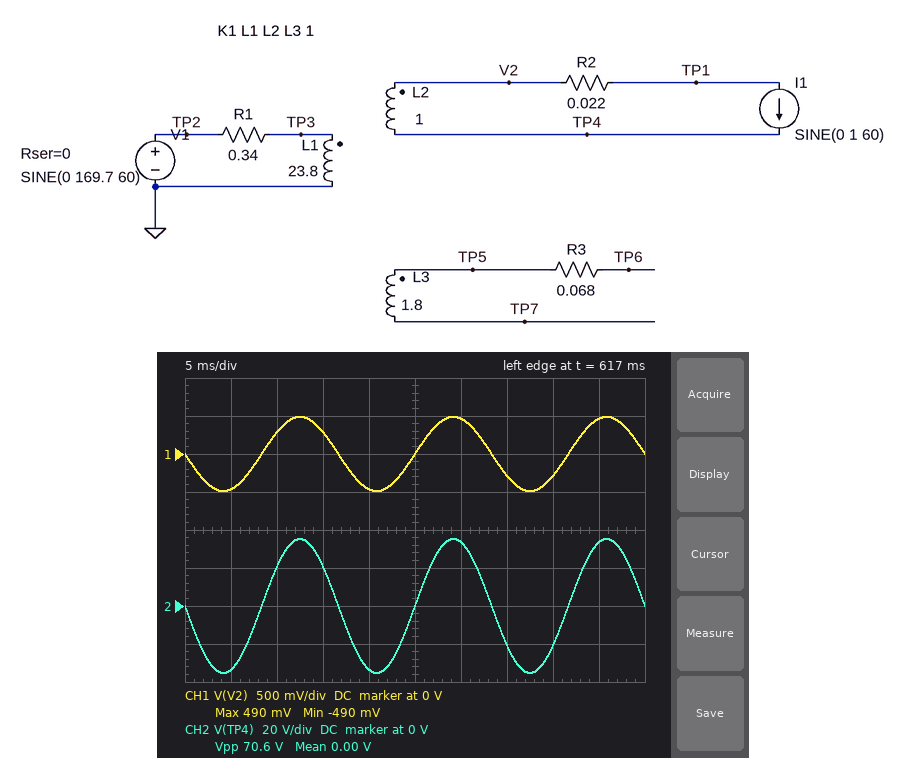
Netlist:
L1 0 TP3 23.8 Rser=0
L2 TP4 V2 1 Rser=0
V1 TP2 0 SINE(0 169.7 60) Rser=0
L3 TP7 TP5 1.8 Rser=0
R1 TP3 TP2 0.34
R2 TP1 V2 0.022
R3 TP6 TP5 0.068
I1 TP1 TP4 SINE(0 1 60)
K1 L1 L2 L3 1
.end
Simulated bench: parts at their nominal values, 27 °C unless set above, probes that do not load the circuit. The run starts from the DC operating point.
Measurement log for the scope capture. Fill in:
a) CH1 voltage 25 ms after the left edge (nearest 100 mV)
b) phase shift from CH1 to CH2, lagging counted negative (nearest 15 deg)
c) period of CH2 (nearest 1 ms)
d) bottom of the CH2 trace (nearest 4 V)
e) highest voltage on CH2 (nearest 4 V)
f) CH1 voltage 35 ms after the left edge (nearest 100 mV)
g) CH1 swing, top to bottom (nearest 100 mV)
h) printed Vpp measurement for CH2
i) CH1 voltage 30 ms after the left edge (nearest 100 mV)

0 V
0 deg
17 ms
-36 V
36 V
-300 mV
1.0 V
70.6 V
500 mV
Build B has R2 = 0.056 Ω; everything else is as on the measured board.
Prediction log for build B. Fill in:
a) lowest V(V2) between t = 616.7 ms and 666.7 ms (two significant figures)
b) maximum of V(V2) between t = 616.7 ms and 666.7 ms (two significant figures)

-470 mV
470 mV
